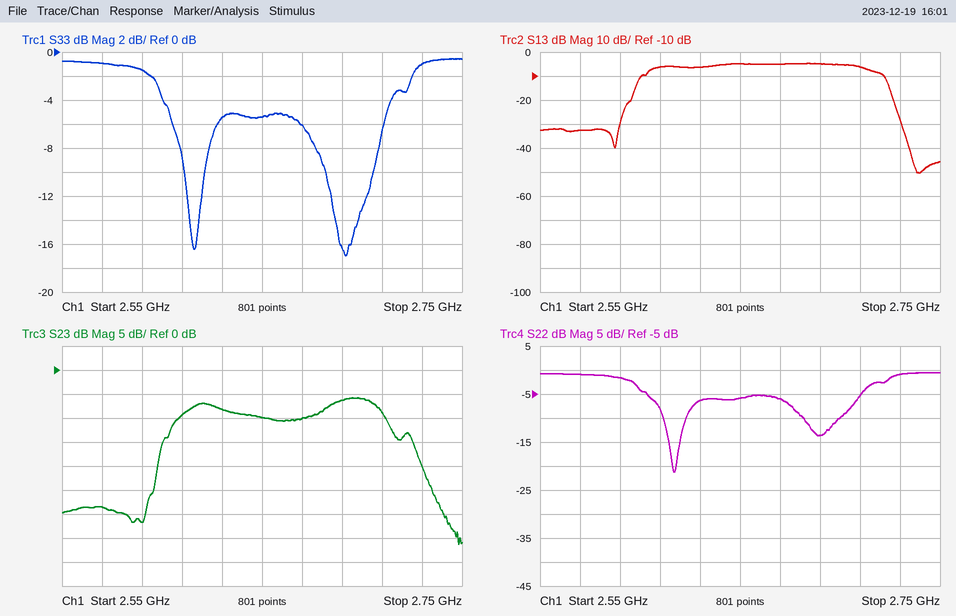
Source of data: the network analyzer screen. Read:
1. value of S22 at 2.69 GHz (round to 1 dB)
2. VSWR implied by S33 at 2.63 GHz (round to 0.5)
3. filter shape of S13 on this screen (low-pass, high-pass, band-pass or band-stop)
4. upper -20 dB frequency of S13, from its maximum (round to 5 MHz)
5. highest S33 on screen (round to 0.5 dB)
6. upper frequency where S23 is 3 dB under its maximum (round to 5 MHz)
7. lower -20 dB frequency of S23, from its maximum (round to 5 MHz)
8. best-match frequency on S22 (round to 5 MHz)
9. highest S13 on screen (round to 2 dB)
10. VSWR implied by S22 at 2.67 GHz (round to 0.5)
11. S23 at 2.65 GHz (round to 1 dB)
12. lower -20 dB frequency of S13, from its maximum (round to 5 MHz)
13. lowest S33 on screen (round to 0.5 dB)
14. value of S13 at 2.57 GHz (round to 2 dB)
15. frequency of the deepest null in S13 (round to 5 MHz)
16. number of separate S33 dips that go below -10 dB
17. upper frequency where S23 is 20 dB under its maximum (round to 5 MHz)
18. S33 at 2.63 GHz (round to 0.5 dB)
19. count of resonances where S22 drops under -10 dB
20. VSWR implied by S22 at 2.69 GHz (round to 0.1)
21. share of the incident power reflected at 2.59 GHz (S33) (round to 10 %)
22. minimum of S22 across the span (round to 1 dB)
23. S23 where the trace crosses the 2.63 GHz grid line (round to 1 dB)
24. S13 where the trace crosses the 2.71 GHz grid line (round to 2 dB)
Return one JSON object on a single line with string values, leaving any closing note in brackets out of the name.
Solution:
{"value of S22 at 2.69 GHz": "-14 dB", "VSWR implied by S33 at 2.63 GHz": "3.5", "filter shape of S13 on this screen": "band-pass", "upper -20 dB frequency of S13, from its maximum": "2.730 GHz", "highest S33 on screen": "-0.5 dB", "upper frequency where S23 is 3 dB under its maximum": "2.710 GHz", "lower -20 dB frequency of S23, from its maximum": "2.595 GHz", "best-match frequency on S22": "2.615 GHz", "highest S13 on screen": "-4 dB", "VSWR implied by S22 at 2.67 GHz": "3.0", "S23 at 2.65 GHz": "-10 dB", "lower -20 dB frequency of S13, from its maximum": "2.590 GHz", "lowest S33 on screen": "-17.0 dB", "value of S13 at 2.57 GHz": "-32 dB", "frequency of the deepest null in S13": "2.740 GHz", "number of separate S33 dips that go below -10 dB": "2", "upper frequency where S23 is 20 dB under its maximum": "2.735 GHz", "S33 at 2.63 GHz": "-5.5 dB", "count of resonances where S22 drops under -10 dB": "2", "VSWR implied by S22 at 2.69 GHz": "1.5", "share of the incident power reflected at 2.59 GHz (S33)": "70 %", "minimum of S22 across the span": "-21 dB", "S23 where the trace crosses the 2.63 GHz grid line": "-8 dB", "S13 where the trace crosses the 2.71 GHz grid line": "-6 dB"}
